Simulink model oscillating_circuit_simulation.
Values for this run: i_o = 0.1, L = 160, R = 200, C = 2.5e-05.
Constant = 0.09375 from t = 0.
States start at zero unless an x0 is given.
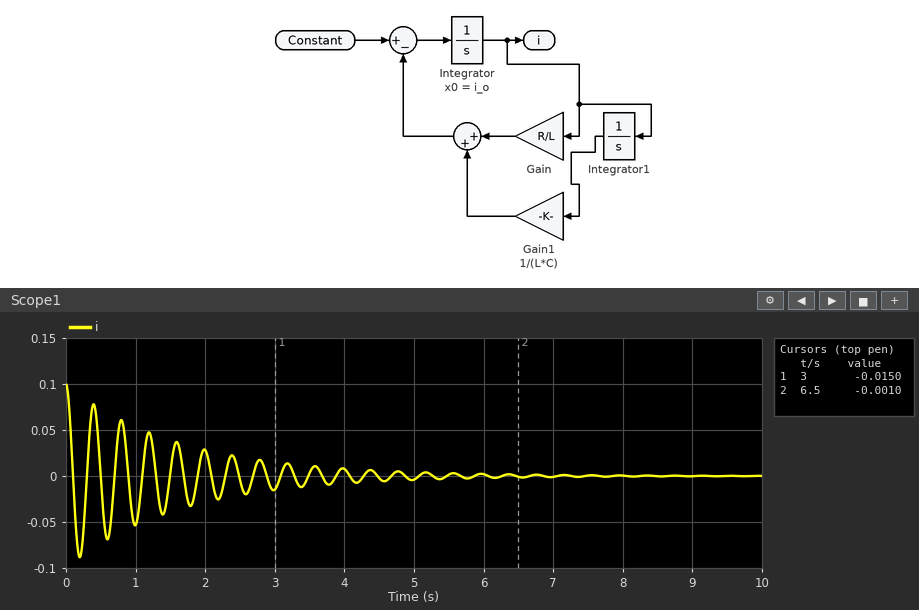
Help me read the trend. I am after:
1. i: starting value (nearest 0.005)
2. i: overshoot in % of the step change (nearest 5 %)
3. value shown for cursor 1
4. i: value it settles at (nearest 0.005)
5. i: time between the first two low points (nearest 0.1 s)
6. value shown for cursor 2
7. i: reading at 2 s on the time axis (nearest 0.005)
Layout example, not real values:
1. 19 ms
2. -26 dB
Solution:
1. 0.100
2. 90 %
3. -0.0150
4. 0.000
5. 0.4 s
6. -0.0010
7. 0.030
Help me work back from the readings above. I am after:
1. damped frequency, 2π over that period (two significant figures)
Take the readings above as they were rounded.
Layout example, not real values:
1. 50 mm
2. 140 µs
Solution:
1. 16 rad/s
